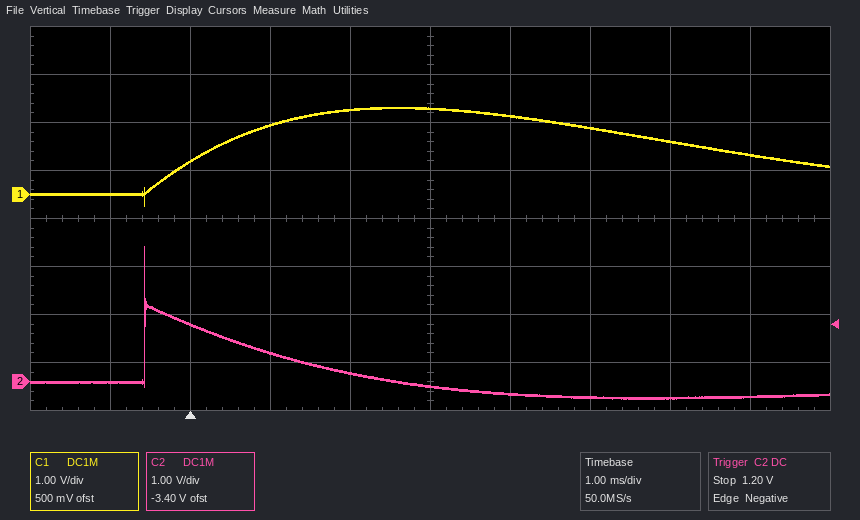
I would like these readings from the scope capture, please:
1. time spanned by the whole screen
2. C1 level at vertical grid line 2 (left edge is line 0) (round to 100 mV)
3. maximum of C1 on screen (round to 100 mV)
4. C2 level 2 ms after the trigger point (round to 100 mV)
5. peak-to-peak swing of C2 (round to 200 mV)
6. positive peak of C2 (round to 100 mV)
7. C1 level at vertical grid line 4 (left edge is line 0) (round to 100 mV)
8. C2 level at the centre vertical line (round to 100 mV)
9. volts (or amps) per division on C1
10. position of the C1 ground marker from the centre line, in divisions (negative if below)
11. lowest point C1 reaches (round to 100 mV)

10 ms
700 mV
1.8 V
200 mV
3.2 V
2.8 V
1.8 V
-100 mV
1 V
+0.5 div
-200 mV
